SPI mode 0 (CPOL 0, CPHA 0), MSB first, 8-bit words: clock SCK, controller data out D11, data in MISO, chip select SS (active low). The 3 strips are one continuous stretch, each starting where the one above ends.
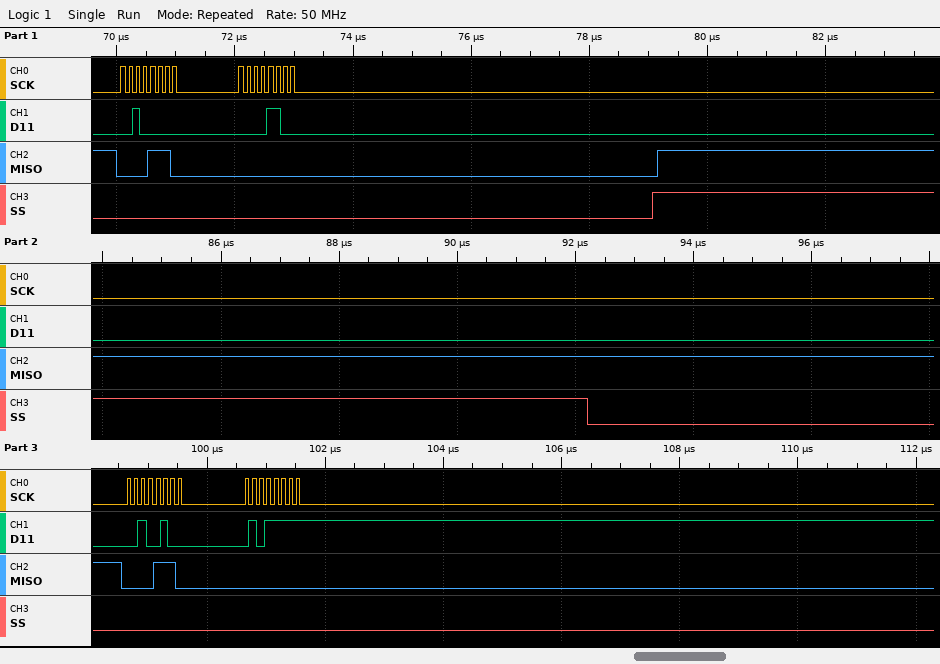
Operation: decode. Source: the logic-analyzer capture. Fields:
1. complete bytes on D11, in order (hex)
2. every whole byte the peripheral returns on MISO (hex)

0x20 0x0C 0x24 0x5F
0x0E 0x00 0x0E 0x00
